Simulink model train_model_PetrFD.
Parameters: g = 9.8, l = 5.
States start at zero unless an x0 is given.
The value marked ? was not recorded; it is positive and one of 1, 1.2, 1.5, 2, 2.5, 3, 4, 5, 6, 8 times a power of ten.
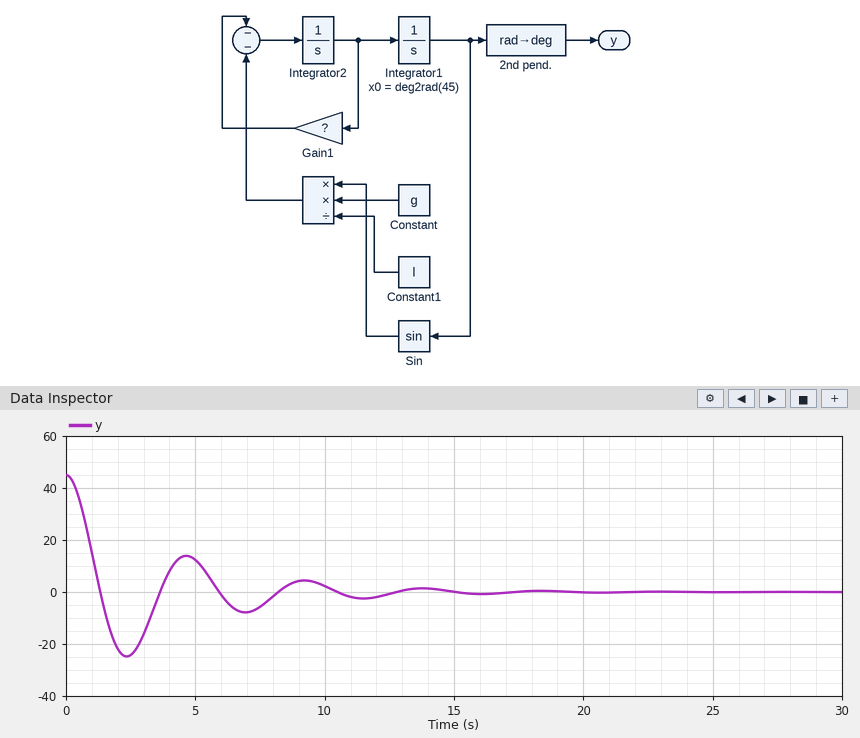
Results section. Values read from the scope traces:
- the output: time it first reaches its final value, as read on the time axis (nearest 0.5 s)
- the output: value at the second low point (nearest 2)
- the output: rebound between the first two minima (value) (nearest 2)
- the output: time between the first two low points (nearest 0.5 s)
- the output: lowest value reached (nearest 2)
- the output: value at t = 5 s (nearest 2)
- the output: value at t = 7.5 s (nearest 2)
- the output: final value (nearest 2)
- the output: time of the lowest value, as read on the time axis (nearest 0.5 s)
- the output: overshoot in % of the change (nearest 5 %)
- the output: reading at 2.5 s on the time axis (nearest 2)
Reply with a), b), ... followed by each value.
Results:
a) 1.5 s
b) -8
c) 14
d) 4.5 s
e) -24
f) 12
g) -6
h) 0
i) 2.5 s
j) 55 %
k) -24
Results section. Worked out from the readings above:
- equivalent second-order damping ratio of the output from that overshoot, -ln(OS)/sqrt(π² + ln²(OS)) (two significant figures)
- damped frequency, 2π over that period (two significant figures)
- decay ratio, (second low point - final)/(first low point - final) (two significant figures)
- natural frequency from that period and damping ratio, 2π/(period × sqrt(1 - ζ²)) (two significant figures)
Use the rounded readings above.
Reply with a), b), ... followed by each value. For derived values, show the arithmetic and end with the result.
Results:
a) ln(0.55) = -0.598; 0.598 / sqrt(9.870 + 0.357) = 0.19
b) 2π / 4.5 = 1.4 rad/s
c) (-8 - 0) / (-24 - 0) = 0.33
d) 2π / (4.5 × sqrt(1 - 0.19²)) = 1.4 rad/s
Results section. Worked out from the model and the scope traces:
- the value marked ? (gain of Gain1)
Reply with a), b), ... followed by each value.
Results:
a) 0.5
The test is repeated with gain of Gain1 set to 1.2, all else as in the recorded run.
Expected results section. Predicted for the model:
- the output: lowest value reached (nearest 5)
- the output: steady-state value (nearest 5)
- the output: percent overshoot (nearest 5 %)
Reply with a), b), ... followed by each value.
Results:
a) -10
b) 0
c) 20 %
